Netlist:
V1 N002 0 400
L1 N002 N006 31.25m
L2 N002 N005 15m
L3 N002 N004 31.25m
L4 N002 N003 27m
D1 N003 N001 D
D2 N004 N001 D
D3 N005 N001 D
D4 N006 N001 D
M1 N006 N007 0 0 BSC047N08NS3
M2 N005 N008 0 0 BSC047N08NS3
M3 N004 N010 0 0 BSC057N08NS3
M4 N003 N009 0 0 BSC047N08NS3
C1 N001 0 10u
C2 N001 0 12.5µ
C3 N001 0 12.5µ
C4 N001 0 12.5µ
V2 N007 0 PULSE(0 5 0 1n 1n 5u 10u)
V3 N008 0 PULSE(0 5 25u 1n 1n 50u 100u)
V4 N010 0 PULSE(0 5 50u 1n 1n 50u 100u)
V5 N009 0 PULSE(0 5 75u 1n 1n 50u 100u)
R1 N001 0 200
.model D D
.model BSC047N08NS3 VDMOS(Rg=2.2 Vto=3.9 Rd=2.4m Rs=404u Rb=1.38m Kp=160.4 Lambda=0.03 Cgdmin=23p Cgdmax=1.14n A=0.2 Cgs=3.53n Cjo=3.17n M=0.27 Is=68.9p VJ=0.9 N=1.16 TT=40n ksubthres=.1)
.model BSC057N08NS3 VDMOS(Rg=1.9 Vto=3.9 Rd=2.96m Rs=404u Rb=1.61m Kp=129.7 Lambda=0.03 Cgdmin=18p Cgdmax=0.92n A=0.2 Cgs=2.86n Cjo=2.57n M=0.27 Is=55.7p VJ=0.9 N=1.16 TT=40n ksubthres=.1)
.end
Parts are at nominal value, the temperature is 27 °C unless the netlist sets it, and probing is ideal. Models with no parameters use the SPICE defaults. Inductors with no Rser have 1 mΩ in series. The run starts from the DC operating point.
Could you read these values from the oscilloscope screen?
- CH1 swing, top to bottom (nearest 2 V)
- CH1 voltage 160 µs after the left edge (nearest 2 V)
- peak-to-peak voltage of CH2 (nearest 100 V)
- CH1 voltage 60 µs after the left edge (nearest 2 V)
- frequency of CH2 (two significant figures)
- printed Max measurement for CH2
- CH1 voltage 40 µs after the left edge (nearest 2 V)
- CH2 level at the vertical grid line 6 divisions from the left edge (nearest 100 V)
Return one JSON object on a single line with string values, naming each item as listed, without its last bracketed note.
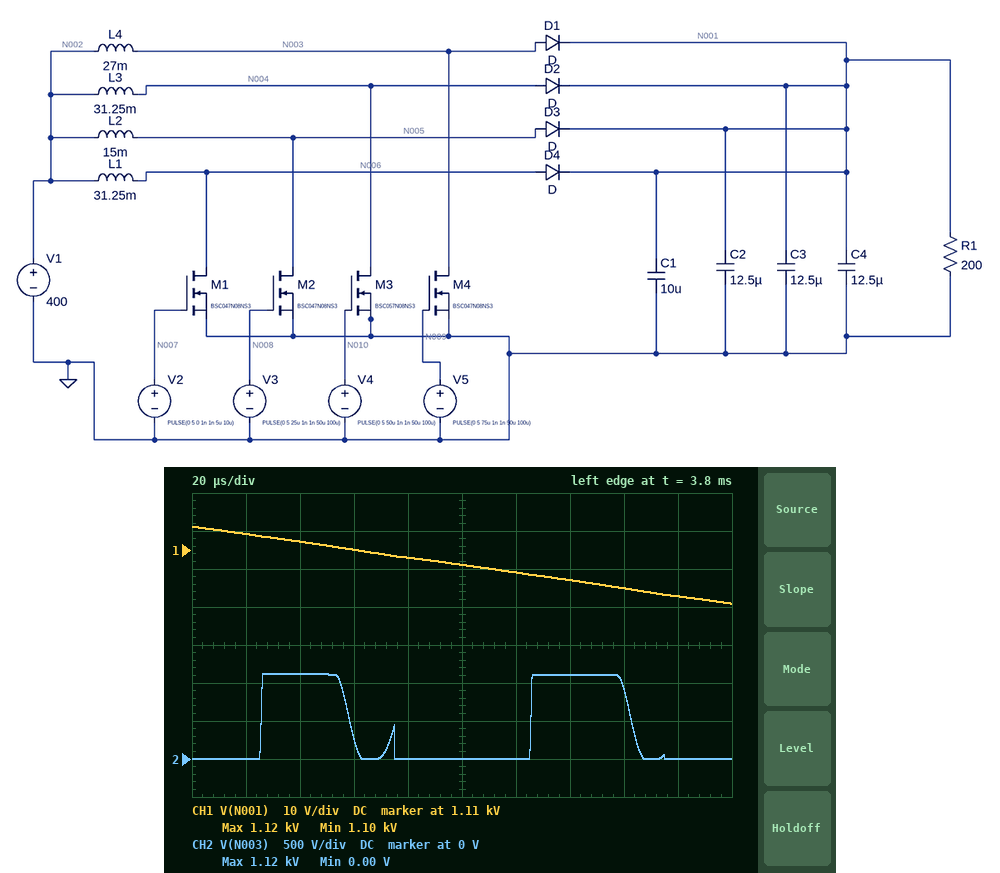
{"CH1 swing, top to bottom": "20 V", "CH1 voltage 160 µs after the left edge": "1.100 kV", "peak-to-peak voltage of CH2": "1.1 kV", "CH1 voltage 60 µs after the left edge": "1.110 kV", "frequency of CH2": "10 kHz", "printed Max measurement for CH2": "1.12 kV", "CH1 voltage 40 µs after the left edge": "1.112 kV", "CH2 level at the vertical grid line 6 divisions from the left edge": "0 V"}
